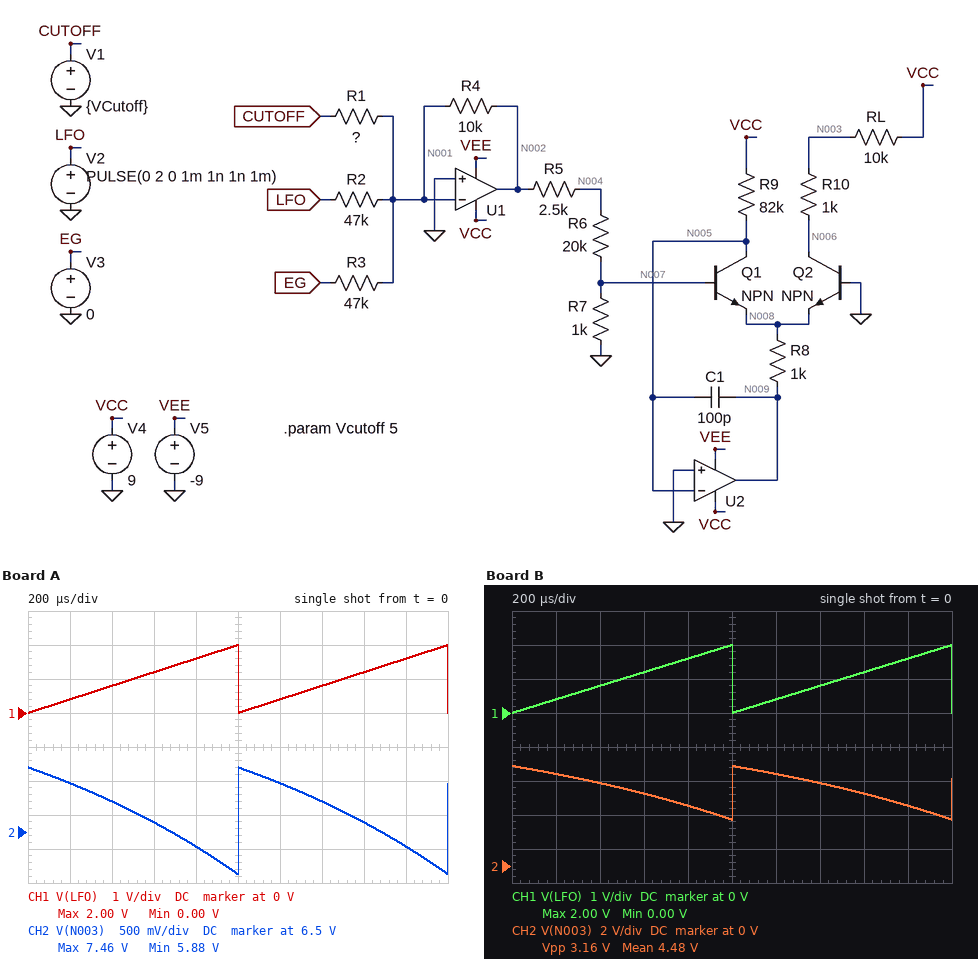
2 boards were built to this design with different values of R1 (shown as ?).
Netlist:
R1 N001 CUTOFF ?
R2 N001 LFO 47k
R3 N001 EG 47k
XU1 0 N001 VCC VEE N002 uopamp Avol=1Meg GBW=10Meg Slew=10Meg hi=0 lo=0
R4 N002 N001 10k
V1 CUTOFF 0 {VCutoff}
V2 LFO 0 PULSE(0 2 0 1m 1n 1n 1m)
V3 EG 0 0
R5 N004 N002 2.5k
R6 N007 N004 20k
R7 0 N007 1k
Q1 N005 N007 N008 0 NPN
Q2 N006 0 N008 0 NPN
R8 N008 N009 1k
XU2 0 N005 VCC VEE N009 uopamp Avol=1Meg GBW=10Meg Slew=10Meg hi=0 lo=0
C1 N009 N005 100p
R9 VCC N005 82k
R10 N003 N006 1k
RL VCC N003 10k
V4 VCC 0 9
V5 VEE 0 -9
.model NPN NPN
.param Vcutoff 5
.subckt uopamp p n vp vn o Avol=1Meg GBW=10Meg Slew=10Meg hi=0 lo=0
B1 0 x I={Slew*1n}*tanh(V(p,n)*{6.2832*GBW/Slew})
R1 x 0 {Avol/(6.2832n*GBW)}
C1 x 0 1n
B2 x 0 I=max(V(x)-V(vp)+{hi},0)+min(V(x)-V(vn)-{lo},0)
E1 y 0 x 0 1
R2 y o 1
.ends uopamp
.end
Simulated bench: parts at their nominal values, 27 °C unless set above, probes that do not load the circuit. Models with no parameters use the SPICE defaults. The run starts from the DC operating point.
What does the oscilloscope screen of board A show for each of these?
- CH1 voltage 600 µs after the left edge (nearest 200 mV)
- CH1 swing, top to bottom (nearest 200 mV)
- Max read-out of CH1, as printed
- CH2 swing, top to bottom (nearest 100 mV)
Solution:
1.2 V
2.0 V
2.00 V
1.6 V
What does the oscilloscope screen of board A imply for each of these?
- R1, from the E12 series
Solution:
270 kΩ
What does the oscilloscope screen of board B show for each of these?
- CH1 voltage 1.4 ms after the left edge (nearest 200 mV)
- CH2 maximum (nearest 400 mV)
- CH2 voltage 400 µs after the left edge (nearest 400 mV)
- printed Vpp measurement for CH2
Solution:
800 mV
6.0 V
4.8 V
3.16 V
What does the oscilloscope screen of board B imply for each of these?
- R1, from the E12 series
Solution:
82 kΩ
